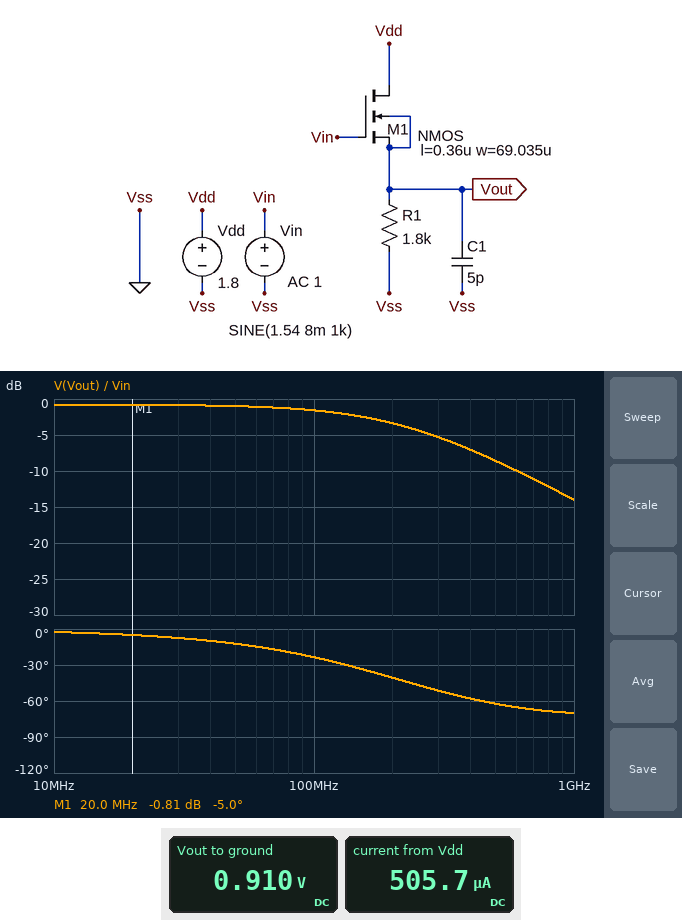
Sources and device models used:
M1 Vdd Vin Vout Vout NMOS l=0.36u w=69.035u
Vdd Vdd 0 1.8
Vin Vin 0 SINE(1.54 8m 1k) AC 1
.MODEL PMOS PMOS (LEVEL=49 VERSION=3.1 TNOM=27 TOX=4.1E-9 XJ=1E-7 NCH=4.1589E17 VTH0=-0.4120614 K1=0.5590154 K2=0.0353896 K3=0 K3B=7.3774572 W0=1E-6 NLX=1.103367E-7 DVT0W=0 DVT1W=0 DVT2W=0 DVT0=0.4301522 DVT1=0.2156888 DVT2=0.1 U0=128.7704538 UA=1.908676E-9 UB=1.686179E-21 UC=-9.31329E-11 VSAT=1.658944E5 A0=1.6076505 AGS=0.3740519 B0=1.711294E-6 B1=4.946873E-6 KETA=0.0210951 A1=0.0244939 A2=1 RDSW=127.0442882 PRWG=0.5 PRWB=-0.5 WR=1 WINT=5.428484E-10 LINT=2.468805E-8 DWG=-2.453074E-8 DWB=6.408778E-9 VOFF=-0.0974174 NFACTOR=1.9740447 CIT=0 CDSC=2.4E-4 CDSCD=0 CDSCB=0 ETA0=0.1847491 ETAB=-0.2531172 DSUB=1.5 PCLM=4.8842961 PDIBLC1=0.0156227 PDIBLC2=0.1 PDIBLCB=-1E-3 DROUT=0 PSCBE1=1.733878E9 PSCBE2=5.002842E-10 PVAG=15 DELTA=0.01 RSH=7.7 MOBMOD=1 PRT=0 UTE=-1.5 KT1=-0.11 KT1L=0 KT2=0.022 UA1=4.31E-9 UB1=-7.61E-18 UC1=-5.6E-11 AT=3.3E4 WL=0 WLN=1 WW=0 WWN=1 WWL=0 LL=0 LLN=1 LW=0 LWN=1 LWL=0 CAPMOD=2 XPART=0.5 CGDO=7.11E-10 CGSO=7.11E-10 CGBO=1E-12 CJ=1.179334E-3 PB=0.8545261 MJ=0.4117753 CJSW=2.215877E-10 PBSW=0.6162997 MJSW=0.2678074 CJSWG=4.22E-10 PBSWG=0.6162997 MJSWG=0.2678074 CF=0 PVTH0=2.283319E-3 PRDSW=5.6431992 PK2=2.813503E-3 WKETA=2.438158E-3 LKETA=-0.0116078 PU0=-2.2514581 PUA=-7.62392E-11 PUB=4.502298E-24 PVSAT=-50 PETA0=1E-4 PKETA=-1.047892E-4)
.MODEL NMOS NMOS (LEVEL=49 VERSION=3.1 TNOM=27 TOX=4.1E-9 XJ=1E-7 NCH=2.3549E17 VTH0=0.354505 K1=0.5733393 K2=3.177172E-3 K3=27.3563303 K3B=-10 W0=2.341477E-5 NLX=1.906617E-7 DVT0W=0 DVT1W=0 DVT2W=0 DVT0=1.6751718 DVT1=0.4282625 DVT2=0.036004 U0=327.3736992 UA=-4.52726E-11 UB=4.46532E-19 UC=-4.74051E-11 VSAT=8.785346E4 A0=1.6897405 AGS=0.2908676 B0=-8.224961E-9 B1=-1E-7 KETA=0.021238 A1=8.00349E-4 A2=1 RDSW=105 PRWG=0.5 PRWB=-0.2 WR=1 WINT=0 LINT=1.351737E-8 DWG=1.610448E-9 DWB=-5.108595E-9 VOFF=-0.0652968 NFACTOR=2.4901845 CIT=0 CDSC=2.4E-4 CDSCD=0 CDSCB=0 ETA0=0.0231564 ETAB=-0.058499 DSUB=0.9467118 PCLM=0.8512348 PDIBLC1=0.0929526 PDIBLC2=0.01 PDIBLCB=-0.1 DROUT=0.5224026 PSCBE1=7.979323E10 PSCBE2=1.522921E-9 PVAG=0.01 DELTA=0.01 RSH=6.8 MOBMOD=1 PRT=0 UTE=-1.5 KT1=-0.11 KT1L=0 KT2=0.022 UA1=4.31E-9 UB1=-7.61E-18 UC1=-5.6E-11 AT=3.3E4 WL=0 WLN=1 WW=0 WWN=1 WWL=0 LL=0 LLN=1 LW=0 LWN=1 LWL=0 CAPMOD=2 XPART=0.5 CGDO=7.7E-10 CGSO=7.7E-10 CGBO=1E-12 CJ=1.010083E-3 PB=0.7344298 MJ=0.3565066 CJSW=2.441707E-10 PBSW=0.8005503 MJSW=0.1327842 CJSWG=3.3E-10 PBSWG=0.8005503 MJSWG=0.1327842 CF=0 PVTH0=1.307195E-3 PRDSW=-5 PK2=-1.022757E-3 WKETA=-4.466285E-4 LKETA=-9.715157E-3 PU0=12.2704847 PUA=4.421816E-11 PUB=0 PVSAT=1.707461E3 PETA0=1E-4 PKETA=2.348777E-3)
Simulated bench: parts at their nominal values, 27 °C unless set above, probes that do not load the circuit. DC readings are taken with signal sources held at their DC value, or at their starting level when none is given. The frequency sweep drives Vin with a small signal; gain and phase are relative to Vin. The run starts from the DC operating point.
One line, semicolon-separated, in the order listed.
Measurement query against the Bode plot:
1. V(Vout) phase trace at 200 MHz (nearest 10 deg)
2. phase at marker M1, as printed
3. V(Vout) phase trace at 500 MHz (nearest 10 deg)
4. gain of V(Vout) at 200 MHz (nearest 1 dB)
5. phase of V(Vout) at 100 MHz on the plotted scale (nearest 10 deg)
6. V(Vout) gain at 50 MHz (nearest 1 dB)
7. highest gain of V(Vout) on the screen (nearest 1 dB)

-40 deg; -5.0 deg; -60 deg; -3 dB; -20 deg; -1 dB; -1 dB
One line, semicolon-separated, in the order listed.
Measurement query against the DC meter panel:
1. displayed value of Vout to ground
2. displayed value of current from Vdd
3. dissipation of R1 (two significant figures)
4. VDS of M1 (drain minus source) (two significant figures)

0.910 V; 505.7 µA; 460 µW; 890 mV
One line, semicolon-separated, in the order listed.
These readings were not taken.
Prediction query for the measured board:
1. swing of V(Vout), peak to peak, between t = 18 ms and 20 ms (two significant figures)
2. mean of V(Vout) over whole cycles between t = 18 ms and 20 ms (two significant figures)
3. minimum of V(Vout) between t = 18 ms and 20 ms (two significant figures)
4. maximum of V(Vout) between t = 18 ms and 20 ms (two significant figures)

15 mV; 910 mV; 900 mV; 920 mV
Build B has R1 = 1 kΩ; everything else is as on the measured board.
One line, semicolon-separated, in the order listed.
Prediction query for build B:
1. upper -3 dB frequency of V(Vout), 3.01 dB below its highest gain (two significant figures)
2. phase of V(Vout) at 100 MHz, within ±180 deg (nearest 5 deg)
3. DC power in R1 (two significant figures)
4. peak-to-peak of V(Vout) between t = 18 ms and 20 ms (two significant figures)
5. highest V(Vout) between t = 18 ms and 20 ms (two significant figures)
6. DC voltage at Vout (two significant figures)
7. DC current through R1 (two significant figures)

300 MHz; -20 deg; 750 µW; 14 mV; 870 mV; 860 mV; 860 µA
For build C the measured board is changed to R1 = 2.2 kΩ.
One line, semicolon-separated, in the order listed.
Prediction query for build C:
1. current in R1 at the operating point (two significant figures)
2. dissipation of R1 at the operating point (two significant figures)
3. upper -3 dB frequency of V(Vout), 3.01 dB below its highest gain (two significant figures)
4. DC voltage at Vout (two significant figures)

420 µA; 390 µW; 200 MHz; 920 mV
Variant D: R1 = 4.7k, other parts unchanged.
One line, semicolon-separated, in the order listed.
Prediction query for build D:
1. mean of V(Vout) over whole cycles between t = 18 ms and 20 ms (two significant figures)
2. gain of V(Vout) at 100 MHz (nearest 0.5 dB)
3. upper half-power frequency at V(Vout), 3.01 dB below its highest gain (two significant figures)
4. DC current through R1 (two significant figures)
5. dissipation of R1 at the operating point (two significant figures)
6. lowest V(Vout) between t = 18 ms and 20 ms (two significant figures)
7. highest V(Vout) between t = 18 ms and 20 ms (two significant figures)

970 mV; -3.0 dB; 120 MHz; 210 µA; 200 µW; 960 mV; 980 mV
